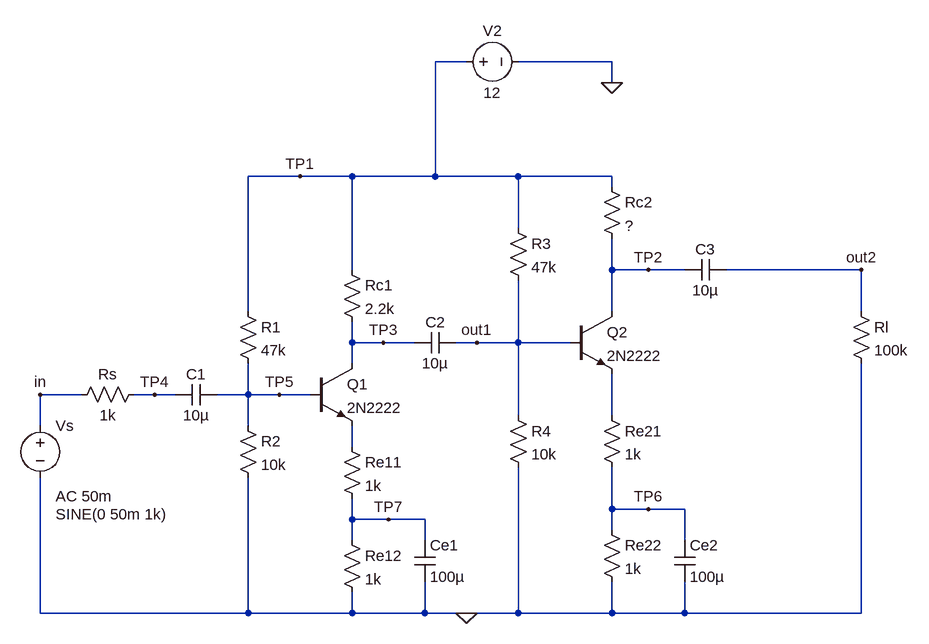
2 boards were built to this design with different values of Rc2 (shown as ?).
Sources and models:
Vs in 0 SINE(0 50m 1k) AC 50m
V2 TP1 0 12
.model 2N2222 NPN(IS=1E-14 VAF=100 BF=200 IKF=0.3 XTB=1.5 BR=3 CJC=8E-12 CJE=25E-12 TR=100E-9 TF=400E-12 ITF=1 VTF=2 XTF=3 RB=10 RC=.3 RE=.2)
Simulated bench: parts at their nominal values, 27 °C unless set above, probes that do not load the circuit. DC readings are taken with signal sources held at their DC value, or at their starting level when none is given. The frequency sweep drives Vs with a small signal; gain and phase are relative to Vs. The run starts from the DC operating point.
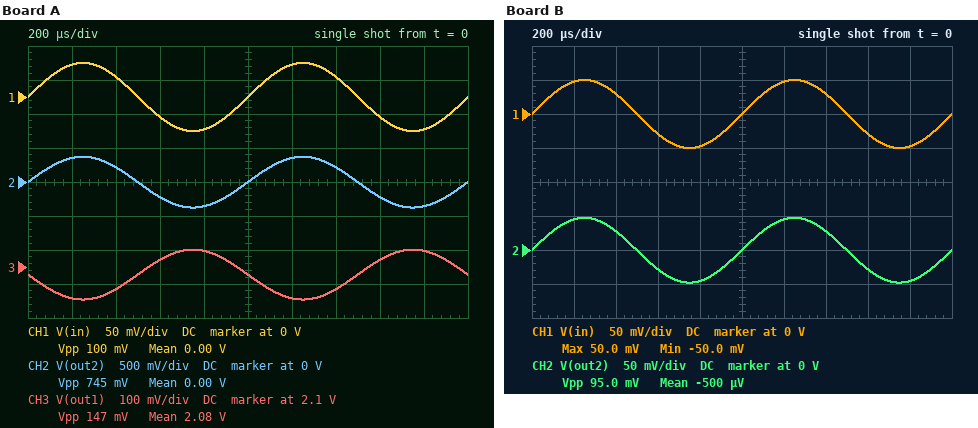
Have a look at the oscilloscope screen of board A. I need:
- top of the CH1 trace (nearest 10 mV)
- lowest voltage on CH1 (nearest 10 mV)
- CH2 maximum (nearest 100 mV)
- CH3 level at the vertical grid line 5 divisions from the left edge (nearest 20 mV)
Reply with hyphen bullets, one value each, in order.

- 50 mV
- -50 mV
- 400 mV
- 2.08 V
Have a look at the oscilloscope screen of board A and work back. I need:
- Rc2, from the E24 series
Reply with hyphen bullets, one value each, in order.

- 5.6 kΩ
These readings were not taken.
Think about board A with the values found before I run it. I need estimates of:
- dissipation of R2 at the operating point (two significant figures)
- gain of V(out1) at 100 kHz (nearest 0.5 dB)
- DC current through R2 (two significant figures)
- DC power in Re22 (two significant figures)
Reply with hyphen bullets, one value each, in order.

- 430 µW
- 3.5 dB
- 210 µA
- 510 µW
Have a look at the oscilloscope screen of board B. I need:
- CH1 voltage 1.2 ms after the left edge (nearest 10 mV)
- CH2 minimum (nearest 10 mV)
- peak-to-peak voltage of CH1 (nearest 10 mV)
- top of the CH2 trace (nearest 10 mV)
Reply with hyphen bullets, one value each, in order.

- 50 mV
- -50 mV
- 100 mV
- 50 mV
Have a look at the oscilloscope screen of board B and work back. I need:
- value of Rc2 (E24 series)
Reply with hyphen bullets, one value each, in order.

- 680 Ω
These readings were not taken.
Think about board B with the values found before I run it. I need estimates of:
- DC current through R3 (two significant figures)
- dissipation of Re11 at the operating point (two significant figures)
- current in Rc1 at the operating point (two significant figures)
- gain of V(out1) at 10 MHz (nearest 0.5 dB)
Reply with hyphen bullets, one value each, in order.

- 210 µA
- 510 µW
- 710 µA
- -2.5 dB
